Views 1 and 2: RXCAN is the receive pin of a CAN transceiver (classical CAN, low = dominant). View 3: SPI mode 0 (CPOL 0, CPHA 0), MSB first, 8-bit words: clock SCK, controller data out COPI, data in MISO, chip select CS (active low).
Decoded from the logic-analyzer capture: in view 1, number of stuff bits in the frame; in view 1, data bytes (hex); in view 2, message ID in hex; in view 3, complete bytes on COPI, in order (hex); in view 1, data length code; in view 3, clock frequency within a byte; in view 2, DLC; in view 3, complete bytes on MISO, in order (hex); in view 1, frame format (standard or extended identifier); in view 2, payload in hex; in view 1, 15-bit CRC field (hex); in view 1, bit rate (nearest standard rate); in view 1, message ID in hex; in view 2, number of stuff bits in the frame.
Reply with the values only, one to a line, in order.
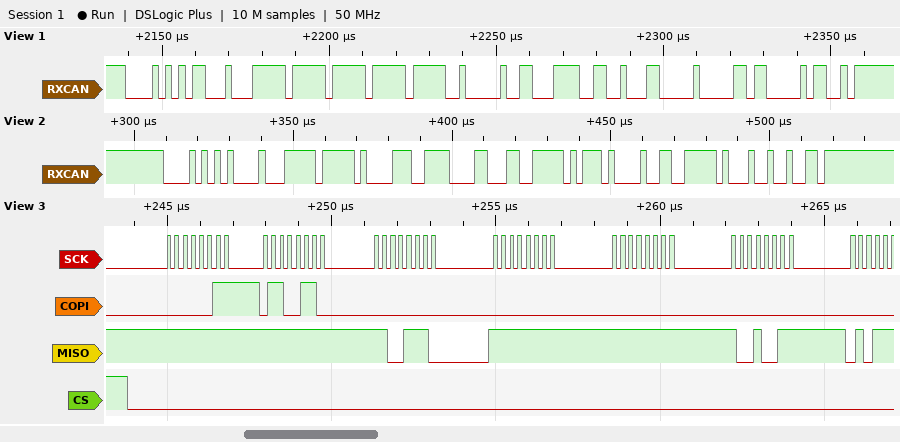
9
FF FF FF A0 31 E6 46 00
0x0AA
03 66 00 00 00 00
8
4 MHz
8
FF FF CE FF FF 93
standard
FF E1 CF 0C 67 EE 84 CF
0x2C0C
500 kbit/s
0x0AB
4
